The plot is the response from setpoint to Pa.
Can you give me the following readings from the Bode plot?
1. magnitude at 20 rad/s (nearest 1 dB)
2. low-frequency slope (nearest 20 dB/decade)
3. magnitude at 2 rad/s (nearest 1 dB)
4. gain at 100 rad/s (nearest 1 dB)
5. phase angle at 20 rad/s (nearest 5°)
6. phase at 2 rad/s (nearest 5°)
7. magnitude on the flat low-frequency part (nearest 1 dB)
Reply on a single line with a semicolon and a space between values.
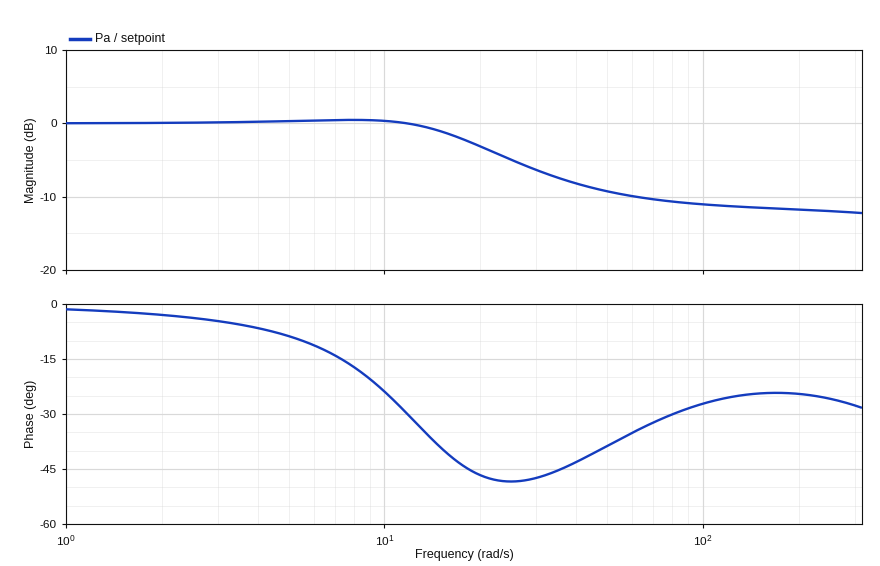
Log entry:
-3 dB; 0 dB/decade; 0 dB; -11 dB; -45°; -5°; 0 dB
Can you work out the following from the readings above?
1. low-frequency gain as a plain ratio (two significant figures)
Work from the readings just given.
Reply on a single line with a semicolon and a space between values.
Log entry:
1.0
